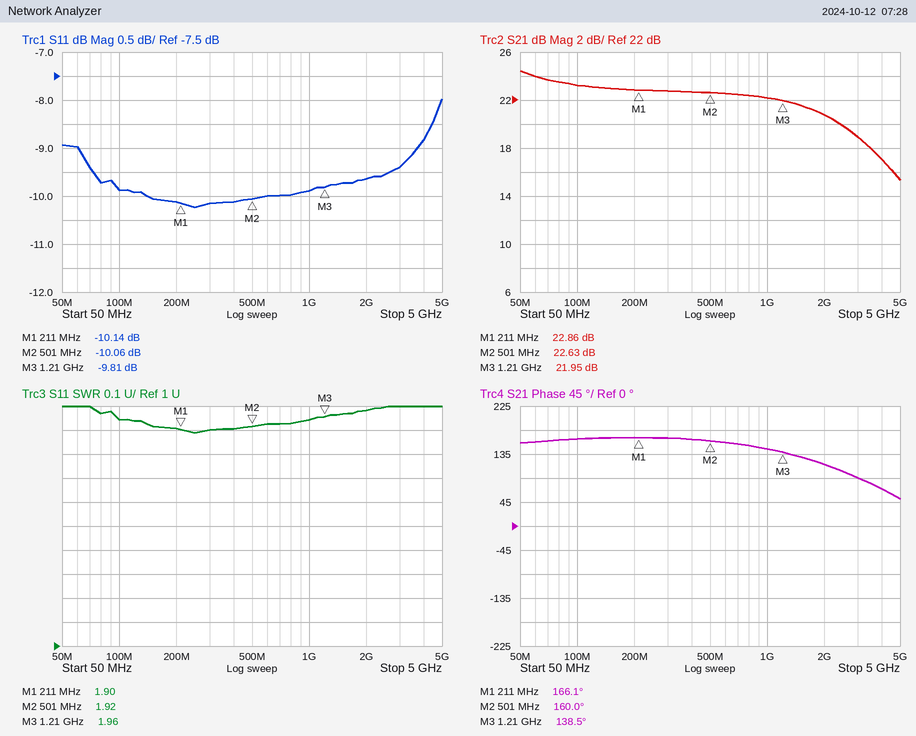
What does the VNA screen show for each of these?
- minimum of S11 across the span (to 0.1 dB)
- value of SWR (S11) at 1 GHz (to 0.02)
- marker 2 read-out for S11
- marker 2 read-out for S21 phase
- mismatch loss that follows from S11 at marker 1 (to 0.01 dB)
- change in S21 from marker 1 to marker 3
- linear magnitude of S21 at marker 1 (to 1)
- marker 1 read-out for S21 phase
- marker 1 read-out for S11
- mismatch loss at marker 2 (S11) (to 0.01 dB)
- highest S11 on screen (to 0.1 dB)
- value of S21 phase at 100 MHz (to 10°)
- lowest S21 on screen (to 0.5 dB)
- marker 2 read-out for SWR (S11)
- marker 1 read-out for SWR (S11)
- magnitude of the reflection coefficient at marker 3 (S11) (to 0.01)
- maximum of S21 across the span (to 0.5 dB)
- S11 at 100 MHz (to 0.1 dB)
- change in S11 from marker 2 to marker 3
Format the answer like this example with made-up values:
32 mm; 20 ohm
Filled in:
-10.2 dB; 1.94; -10.06 dB; 160.0°; 0.44 dB; -0.91 dB; 14; 166.1°; -10.14 dB; 0.45 dB; -8.0 dB; 160°; 15.5 dB; 1.92; 1.90; 0.32; 24.5 dB; -9.9 dB; 0.25 dB
